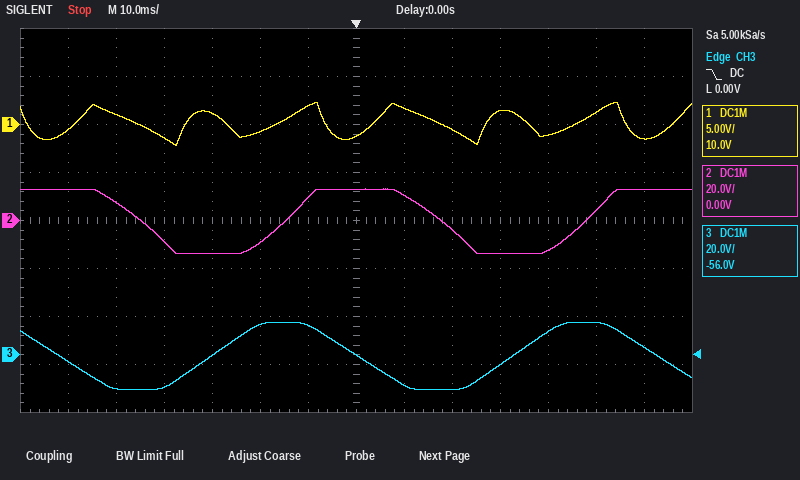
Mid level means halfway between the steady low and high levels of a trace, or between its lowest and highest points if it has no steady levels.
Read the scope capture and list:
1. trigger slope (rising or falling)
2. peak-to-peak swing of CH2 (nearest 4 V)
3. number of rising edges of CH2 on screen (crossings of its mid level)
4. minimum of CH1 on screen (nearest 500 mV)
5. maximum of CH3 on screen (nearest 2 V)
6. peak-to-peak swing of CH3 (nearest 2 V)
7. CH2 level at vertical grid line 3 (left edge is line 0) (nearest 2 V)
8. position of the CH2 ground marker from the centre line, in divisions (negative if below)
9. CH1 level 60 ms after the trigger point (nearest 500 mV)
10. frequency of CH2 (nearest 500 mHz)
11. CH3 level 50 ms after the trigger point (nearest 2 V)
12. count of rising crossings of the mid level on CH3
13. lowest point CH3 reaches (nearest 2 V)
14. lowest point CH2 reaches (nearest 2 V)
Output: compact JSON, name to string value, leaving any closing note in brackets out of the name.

{"trigger slope": "falling", "peak-to-peak swing of CH2": "28 V", "number of rising edges of CH2 on screen": "2", "minimum of CH1 on screen": "-2.0 V", "maximum of CH3 on screen": "14 V", "peak-to-peak swing of CH3": "28 V", "CH2 level at vertical grid line 3 (left edge is line 0)": "-8 V", "position of the CH2 ground marker from the centre line, in divisions": "0.0 div", "CH1 level 60 ms after the trigger point": "-1.5 V", "frequency of CH2": "16.0 Hz", "CH3 level 50 ms after the trigger point": "14 V", "count of rising crossings of the mid level on CH3": "2", "lowest point CH3 reaches": "-14 V", "lowest point CH2 reaches": "-14 V"}
